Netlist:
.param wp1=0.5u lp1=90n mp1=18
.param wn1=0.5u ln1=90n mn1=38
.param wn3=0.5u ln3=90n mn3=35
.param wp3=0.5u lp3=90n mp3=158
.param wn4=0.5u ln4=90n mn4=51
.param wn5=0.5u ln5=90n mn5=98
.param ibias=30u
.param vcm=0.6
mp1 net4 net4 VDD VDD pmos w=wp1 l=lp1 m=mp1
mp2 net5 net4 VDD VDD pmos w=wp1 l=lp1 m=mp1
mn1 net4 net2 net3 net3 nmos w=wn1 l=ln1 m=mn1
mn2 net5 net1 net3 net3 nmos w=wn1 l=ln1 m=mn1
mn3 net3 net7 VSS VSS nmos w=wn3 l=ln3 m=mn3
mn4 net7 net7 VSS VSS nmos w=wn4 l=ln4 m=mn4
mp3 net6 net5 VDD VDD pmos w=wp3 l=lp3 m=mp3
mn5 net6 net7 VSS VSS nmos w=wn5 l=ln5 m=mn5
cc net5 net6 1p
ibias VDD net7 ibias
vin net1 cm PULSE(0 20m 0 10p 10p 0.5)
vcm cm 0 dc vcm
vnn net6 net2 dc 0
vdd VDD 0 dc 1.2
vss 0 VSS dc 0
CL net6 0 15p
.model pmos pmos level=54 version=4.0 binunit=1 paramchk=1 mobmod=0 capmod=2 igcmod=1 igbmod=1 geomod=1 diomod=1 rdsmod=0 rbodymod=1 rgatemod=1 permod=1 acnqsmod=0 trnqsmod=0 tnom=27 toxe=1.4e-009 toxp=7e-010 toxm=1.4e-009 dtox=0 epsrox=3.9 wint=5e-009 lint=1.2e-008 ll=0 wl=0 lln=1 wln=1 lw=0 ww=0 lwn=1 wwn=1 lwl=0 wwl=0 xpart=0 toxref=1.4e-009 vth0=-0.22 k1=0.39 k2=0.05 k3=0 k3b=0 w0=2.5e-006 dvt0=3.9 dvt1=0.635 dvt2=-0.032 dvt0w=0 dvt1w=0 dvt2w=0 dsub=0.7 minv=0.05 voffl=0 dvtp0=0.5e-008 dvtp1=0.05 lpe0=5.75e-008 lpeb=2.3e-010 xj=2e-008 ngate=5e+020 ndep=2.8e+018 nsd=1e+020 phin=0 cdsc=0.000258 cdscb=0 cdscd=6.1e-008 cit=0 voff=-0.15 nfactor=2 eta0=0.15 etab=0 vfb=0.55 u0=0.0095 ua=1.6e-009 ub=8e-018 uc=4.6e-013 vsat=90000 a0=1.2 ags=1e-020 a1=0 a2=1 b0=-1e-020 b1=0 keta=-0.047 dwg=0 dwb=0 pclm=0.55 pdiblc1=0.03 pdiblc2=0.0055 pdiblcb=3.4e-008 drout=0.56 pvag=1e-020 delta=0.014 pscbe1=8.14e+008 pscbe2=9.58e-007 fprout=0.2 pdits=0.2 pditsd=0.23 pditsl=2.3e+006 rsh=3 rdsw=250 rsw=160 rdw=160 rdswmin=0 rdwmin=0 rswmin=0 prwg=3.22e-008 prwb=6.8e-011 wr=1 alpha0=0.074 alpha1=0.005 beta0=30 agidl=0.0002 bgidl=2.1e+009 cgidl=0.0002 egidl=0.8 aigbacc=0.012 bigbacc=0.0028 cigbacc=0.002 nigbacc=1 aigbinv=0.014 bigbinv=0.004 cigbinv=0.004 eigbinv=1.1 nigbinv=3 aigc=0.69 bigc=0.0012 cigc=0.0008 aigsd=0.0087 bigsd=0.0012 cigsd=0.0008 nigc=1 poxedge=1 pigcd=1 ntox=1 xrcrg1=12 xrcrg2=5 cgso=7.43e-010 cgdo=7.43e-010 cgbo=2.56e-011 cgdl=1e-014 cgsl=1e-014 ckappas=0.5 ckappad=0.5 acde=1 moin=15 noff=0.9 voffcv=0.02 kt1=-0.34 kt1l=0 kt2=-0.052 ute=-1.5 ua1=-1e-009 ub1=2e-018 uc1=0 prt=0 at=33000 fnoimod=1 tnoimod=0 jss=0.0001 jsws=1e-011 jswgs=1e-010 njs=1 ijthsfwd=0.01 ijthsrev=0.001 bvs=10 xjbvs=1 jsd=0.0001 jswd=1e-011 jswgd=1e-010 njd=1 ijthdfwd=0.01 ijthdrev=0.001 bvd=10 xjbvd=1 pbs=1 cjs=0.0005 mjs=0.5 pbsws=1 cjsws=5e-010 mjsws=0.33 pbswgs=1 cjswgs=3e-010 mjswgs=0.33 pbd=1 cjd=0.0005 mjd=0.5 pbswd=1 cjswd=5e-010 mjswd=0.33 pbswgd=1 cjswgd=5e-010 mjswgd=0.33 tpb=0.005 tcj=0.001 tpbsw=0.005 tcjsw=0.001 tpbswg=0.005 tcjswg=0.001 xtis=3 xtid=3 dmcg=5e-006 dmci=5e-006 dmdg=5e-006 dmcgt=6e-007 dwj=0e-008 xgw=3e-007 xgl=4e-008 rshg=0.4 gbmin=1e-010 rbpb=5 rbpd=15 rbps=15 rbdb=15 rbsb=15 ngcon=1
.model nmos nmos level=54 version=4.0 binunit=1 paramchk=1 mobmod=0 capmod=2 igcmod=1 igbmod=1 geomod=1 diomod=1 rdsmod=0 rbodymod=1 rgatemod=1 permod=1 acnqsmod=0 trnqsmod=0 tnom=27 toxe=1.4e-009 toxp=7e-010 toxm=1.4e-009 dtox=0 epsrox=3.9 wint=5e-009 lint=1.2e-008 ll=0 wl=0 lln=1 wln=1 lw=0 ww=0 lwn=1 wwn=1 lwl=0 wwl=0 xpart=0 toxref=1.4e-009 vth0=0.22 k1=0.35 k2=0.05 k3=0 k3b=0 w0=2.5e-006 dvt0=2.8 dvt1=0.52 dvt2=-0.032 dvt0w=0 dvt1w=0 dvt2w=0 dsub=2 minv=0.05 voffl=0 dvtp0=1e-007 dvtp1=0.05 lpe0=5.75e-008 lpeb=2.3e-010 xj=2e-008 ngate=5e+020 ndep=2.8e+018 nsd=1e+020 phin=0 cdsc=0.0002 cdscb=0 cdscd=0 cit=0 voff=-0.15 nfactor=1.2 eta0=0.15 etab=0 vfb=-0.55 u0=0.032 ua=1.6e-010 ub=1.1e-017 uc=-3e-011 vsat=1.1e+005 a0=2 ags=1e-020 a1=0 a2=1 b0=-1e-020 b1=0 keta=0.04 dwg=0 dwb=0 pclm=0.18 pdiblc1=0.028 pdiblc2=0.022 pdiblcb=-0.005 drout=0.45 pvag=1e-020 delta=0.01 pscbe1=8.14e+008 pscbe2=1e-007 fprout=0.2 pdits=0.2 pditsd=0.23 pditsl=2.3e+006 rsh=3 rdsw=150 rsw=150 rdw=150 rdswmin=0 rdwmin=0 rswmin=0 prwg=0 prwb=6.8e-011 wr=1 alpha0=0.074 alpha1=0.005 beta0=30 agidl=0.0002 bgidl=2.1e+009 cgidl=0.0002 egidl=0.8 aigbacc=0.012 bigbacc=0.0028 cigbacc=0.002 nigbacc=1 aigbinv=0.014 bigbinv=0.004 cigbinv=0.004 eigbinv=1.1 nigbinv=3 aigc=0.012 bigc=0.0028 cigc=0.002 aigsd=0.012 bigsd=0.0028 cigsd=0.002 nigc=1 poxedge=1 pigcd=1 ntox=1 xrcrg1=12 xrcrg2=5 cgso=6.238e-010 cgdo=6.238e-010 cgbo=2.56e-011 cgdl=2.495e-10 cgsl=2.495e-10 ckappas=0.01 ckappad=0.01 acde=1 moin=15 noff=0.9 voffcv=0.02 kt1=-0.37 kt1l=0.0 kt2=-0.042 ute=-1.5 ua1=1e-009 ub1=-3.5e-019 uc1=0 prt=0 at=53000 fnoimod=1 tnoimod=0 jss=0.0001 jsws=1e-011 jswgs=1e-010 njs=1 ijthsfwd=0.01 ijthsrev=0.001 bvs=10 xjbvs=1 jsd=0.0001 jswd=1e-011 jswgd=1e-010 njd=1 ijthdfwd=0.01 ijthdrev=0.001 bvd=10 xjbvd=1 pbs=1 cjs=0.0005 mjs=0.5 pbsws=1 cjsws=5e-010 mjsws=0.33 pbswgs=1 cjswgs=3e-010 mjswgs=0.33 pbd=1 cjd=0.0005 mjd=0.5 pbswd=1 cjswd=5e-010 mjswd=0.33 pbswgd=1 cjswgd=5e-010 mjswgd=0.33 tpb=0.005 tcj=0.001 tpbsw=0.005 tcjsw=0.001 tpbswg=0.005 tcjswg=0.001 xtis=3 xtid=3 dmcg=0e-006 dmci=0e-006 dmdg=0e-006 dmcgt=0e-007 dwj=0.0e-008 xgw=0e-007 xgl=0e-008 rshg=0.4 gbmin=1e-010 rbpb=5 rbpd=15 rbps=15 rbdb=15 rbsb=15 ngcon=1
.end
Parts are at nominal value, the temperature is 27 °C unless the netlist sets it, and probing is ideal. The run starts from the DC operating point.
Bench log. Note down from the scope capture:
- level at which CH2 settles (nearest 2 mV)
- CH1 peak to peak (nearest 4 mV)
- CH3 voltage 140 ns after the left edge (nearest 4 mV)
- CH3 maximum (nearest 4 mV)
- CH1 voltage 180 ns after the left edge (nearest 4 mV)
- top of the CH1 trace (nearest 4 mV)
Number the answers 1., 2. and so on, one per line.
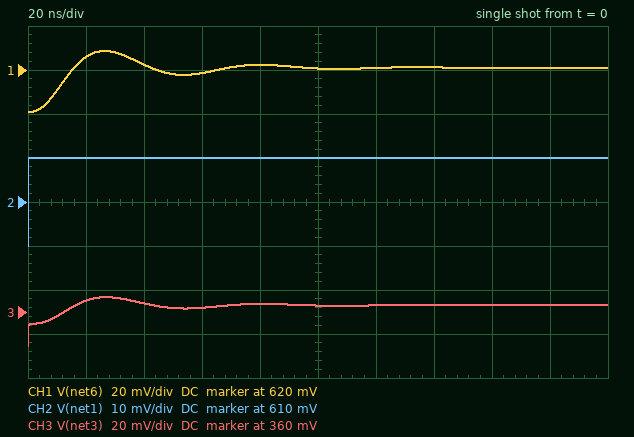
1. 620 mV
2. 28 mV
3. 364 mV
4. 368 mV
5. 620 mV
6. 628 mV
